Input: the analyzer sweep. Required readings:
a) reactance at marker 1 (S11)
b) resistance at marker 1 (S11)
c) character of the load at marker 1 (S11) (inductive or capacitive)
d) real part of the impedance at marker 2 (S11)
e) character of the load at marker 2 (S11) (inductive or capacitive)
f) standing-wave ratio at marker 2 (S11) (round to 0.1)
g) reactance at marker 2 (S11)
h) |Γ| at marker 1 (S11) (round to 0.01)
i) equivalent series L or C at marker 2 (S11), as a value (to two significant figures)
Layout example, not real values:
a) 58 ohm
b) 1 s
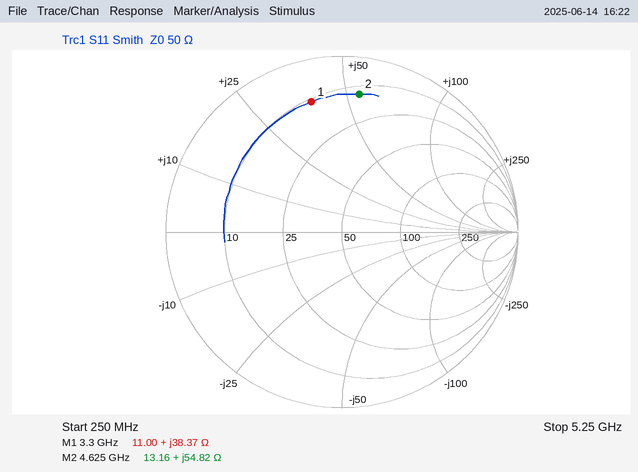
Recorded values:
a) +38.37 Ω
b) 11.00 Ω
c) inductive
d) 13.16 Ω
e) inductive
f) 8.5
g) +54.82 Ω
h) 0.76
i) 1.9 nH
